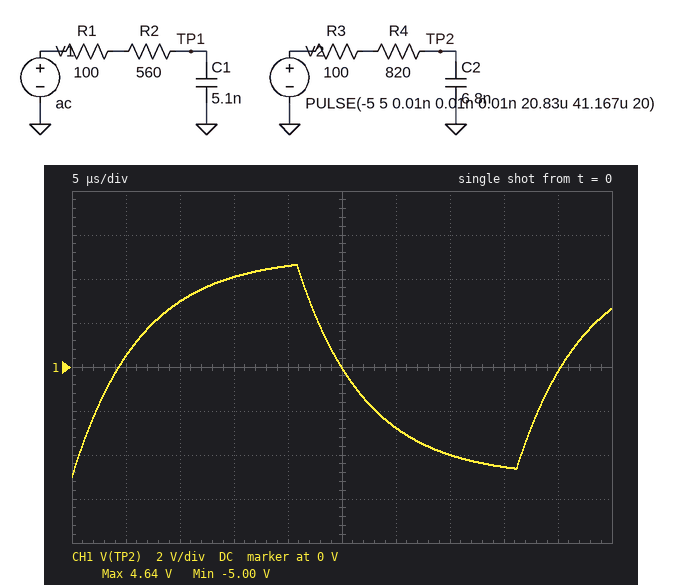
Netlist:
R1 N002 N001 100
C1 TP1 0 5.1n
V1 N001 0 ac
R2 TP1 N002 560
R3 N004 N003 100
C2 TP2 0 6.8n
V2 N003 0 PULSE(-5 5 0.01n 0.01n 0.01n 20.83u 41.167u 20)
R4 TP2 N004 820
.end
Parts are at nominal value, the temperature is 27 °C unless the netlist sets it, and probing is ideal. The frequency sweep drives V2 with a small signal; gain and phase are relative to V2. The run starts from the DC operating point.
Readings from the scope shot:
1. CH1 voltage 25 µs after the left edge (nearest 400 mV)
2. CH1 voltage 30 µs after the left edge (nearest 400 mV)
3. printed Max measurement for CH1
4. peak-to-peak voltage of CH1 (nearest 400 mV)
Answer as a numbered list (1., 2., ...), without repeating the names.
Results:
1. 0 V
2. -2.8 V
3. 4.64 V
4. 9.6 V
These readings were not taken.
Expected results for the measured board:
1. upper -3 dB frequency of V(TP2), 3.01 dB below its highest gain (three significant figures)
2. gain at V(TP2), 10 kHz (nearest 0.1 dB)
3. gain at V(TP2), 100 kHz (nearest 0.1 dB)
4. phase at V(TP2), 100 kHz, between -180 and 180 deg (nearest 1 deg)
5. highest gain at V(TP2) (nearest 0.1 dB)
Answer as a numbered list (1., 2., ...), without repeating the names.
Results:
1. 25.4 kHz
2. -0.6 dB
3. -12.2 dB
4. -76 deg
5. 0 dB
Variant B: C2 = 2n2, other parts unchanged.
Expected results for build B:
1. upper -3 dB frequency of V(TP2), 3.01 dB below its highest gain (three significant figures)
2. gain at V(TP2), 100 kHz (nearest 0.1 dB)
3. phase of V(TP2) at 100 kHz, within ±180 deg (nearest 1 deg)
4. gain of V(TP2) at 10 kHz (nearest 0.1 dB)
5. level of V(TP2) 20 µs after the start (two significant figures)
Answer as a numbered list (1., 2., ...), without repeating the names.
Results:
1. 78.6 kHz
2. -4.2 dB
3. -52 deg
4. -0.1 dB
5. 5.0 V
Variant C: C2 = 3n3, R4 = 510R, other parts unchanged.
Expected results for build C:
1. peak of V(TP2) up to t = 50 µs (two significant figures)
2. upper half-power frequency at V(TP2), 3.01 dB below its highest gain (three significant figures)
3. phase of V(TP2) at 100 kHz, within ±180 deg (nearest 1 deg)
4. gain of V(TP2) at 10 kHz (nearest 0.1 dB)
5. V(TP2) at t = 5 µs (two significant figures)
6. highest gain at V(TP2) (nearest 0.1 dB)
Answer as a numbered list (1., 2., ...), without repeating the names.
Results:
1. 5.0 V
2. 79.1 kHz
3. -52 deg
4. -0.1 dB
5. 4.2 V
6. 0 dB
